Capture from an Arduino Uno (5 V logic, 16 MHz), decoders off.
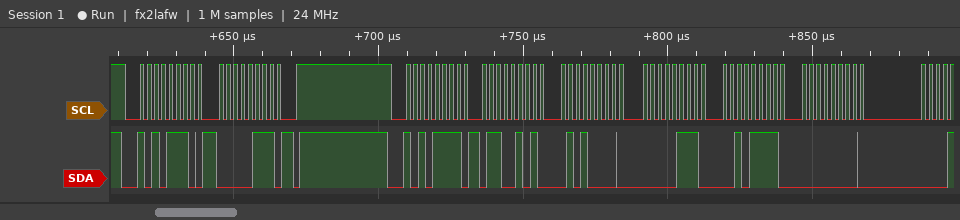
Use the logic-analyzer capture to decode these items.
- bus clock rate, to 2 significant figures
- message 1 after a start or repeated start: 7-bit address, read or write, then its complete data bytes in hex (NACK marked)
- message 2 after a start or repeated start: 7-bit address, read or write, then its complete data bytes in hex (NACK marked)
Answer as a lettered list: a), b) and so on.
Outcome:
a) 400 kHz
b) 0x57 write: 07
c) 0x57 read: 65 50 07 2F 00
